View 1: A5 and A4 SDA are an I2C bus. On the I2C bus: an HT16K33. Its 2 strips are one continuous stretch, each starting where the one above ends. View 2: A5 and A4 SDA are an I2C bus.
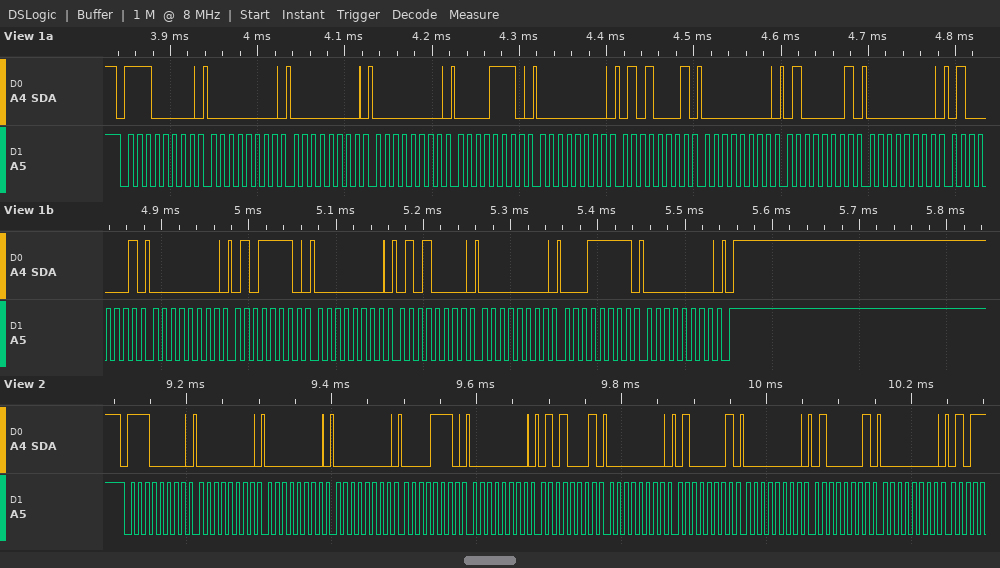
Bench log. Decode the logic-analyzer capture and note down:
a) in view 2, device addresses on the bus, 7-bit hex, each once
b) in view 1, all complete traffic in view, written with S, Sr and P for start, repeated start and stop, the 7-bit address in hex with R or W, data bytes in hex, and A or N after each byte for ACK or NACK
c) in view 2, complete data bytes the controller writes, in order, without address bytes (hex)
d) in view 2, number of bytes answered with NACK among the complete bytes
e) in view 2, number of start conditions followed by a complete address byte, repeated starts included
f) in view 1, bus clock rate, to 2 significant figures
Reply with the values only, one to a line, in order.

0x70
S 70W A 00 A 00 A 00 A 0E A 00 A 51 A 00 A 41 A 00 A 41 A 00 A 5E A 00 A 50 A 00 A 1F A 00 A P
00 00 00 0E 00 51 00 41 00 41 00
0
1
100 kHz
